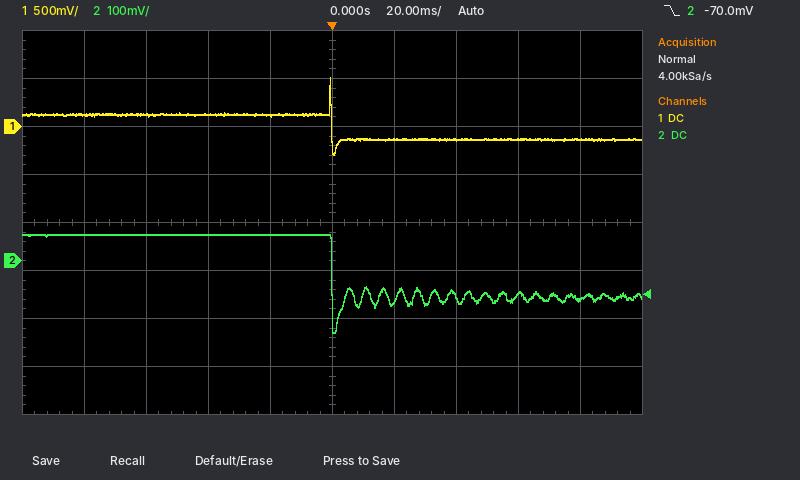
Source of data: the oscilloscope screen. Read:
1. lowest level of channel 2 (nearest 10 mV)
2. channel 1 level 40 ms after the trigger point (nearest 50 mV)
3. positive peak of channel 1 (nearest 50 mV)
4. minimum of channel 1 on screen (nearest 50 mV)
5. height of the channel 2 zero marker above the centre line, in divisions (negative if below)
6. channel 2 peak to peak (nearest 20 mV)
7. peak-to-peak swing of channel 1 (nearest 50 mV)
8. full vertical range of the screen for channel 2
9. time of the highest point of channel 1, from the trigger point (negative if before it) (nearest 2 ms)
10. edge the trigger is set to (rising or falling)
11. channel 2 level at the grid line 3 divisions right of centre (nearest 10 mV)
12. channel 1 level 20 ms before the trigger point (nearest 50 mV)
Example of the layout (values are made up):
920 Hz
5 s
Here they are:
-150 mV
-150 mV
500 mV
-300 mV
-0.8 div
200 mV
800 mV
800 mV
0 ms
falling
-70 mV
100 mV
